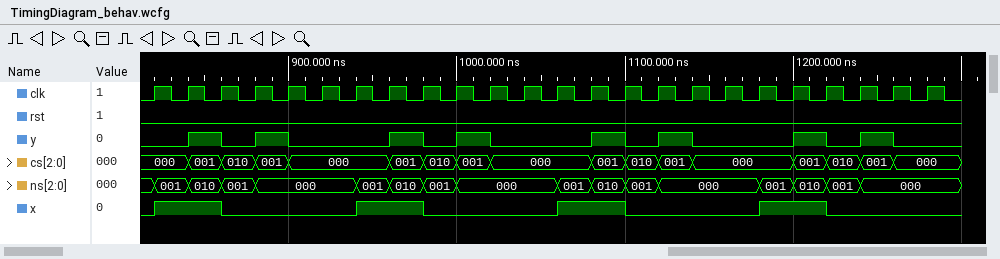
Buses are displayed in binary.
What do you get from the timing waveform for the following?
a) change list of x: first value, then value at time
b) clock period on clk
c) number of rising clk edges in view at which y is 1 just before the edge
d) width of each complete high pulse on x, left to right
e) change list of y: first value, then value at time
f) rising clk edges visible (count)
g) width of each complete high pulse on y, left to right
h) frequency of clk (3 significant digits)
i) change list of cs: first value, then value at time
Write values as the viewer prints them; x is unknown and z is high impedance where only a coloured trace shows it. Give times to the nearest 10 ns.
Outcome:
0, 1 at 820 ns, 0 at 860 ns, 1 at 940 ns, 0 at 980 ns, 1 at 1060 ns, 0 at 1100 ns, 1 at 1180 ns, 0 at 1220 ns
20 ns
8
40 ns, 40 ns, 40 ns, 40 ns
0, 1 at 840 ns, 0 at 860 ns, 1 at 880 ns, 0 at 900 ns, 1 at 960 ns, 0 at 980 ns, 1 at 1000 ns, 0 at 1020 ns, 1 at 1080 ns, 0 at 1100 ns, 1 at 1120 ns, 0 at 1140 ns, 1 at 1200 ns, 0 at 1220 ns, 1 at 1240 ns, 0 at 1260 ns
24
20 ns, 20 ns, 20 ns, 20 ns, 20 ns, 20 ns, 20 ns, 20 ns
50.0 MHz
000, 001 at 840 ns, 010 at 860 ns, 001 at 880 ns, 000 at 900 ns, 001 at 960 ns, 010 at 980 ns, 001 at 1000 ns, 000 at 1020 ns, 001 at 1080 ns, 010 at 1100 ns, 001 at 1120 ns, 000 at 1140 ns, 001 at 1200 ns, 010 at 1220 ns, 001 at 1240 ns, 000 at 1260 ns
